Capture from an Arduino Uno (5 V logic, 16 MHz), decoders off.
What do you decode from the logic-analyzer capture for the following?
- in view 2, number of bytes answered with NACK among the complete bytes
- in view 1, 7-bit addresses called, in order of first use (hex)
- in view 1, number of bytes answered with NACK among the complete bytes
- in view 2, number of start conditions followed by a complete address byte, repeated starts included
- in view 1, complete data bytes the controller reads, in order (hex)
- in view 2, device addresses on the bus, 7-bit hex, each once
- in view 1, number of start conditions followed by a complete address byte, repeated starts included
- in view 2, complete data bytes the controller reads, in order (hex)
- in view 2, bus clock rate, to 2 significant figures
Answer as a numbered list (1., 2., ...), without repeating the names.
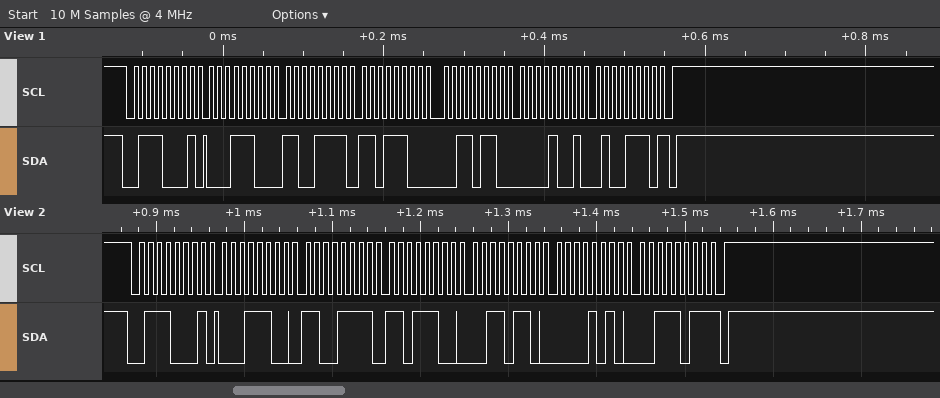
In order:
1. 1
2. 0x38
3. 1
4. 1
5. 1C CF DC 36 09 4E
6. 0x38
7. 1
8. 1C CF DC 36 0A 3B
9. 100 kHz
